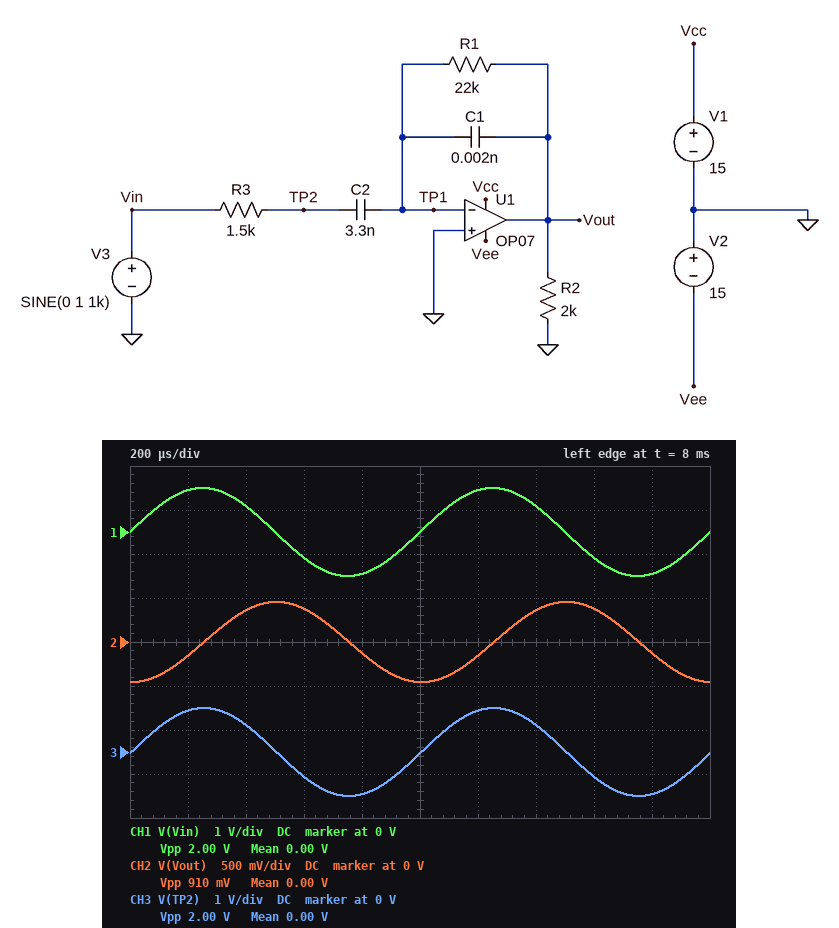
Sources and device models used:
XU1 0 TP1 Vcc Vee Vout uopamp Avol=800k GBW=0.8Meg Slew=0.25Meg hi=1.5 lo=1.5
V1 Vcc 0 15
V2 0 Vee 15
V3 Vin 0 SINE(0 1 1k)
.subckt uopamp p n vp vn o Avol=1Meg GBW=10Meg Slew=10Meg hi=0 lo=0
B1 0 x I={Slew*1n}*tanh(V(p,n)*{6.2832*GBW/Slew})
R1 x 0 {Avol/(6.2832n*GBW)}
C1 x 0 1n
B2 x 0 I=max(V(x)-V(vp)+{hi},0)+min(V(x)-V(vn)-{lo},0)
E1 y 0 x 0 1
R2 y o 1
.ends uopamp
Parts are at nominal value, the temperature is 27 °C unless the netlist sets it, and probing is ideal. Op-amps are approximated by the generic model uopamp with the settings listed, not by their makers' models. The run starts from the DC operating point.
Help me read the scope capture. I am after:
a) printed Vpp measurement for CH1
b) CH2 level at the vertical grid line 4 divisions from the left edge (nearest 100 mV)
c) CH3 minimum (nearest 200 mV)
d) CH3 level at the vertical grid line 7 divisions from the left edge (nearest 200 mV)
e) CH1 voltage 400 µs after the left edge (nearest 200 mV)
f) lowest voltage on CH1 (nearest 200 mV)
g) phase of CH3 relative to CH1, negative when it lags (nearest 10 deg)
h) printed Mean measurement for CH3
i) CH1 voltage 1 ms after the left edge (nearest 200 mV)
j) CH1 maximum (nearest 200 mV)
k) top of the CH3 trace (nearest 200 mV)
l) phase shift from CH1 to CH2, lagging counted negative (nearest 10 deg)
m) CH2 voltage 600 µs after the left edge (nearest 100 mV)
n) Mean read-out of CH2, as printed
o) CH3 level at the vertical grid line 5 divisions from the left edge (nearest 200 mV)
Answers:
2.00 V
-100 mV
-1.0 V
600 mV
600 mV
-1.0 V
0 deg
0.00 V
0 V
1.0 V
1.0 V
-90 deg
400 mV
0.00 V
0 V
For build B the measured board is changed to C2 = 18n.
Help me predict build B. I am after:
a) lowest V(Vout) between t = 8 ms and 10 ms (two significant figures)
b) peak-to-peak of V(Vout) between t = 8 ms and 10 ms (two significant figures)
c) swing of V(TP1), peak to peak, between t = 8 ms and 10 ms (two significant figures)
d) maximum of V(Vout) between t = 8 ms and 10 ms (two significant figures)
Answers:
-2.5 V
4.9 V
6.2 mV
2.5 V
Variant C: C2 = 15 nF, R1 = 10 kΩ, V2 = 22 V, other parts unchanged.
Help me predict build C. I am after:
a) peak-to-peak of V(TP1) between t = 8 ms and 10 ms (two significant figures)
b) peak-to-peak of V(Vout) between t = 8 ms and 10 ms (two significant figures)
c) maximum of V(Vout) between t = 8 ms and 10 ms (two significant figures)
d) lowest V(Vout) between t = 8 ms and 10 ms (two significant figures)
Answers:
2.3 mV
1.9 V
930 mV
-930 mV
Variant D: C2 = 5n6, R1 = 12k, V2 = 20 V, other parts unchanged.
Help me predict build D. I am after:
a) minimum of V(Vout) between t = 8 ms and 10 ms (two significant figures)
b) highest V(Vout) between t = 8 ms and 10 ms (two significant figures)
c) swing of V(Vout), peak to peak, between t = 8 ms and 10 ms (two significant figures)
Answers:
-420 mV
420 mV
840 mV
